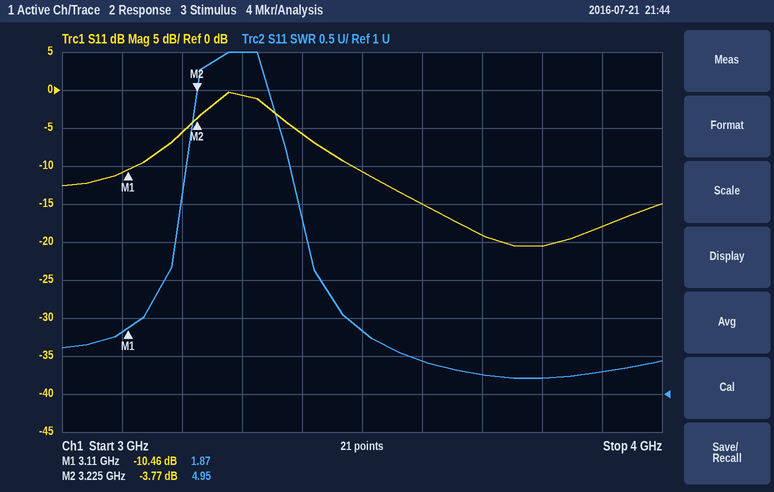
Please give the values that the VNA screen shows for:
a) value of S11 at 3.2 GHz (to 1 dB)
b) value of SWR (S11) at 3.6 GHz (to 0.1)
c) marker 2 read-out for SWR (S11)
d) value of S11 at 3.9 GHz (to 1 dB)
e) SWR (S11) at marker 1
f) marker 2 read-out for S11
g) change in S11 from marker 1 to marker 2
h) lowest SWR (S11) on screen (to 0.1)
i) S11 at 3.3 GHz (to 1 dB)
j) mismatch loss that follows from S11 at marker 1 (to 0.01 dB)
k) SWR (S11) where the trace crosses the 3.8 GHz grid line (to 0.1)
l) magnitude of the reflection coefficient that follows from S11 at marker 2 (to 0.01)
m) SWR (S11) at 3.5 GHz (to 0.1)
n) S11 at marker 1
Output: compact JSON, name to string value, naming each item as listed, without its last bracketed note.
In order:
{"value of S11 at 3.2 GHz": "-6 dB", "value of SWR (S11) at 3.6 GHz": "1.4", "marker 2 read-out for SWR": "4.95", "value of S11 at 3.9 GHz": "-18 dB", "SWR (S11) at marker 1": "1.87", "marker 2 read-out for S11": "-3.77 dB", "change in S11 from marker 1 to marker 2": "6.69 dB", "lowest SWR (S11) on screen": "1.2", "S11 at 3.3 GHz": "-1 dB", "mismatch loss that follows from S11 at marker 1": "0.41 dB", "SWR (S11) where the trace crosses the 3.8 GHz grid line": "1.2", "magnitude of the reflection coefficient that follows from S11 at marker 2": "0.65", "SWR (S11) at 3.5 GHz": "1.8", "S11 at marker 1": "-10.46 dB"}
